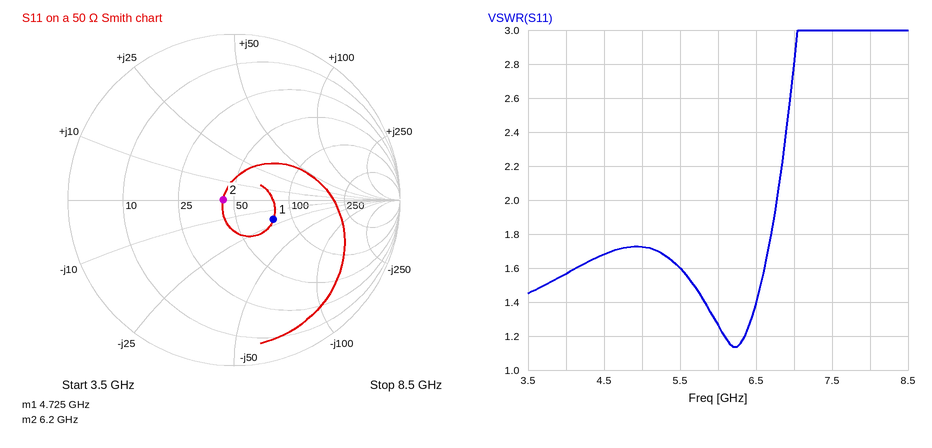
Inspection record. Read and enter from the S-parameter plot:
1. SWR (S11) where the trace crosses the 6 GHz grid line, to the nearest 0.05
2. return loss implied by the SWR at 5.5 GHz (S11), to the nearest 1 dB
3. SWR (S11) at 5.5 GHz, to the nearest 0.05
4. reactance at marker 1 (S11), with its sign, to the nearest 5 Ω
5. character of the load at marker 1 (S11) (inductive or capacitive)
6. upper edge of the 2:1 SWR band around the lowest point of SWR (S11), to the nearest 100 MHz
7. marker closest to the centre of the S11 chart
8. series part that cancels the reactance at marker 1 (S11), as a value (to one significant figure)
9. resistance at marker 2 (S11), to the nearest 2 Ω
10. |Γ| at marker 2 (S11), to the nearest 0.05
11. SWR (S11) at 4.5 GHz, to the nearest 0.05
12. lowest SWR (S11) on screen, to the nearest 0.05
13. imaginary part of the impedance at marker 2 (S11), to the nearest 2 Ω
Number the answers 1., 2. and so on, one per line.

1. 1.25
2. 13 dB
3. 1.60
4. -20 Ω
5. capacitive
6. 6.8 GHz
7. marker 2
8. 700 pH
9. 44 Ω
10. 0.05
11. 1.70
12. 1.15
13. 0 Ω
